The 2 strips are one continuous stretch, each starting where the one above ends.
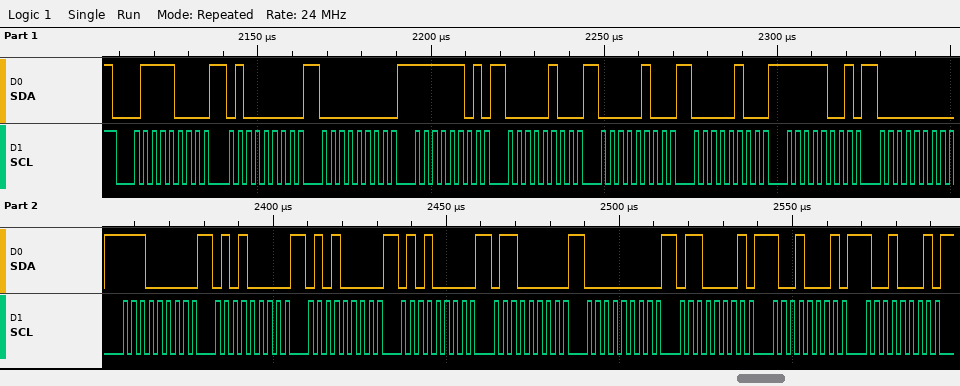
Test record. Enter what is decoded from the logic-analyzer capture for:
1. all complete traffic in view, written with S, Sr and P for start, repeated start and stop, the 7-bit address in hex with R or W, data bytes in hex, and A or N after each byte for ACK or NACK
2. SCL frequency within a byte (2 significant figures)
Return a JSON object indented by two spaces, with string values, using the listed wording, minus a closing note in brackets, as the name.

{
  "all complete traffic in view, written with S, Sr and P for start, repeated start and stop, the 7-bit address in hex with R or W, data bytes in hex, and A or N after each byte for ACK or NACK": "S 3CW A 40 A 00 A FD A 04 A 04 A 04 A F9 A 00 A E0 A 50 A 50 A 50 A 60 A 00 A 61 A 91 A 91 A",
  "SCL frequency within a byte": "400 kHz"
}
